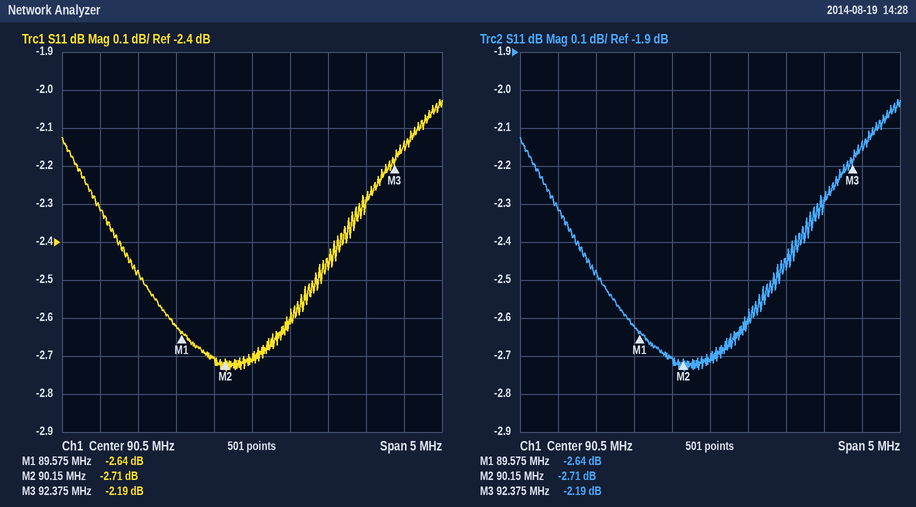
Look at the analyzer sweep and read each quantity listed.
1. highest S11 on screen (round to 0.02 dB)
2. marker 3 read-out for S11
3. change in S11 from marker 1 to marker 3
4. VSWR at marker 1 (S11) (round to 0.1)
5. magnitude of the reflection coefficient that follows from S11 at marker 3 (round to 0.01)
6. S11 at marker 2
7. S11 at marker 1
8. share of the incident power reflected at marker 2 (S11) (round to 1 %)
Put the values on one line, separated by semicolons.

-2.02 dB; -2.19 dB; 0.45 dB; 6.6; 0.78; -2.71 dB; -2.64 dB; 54 %
